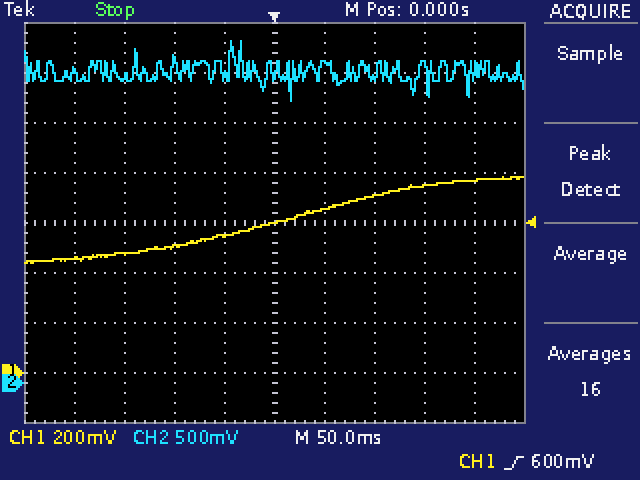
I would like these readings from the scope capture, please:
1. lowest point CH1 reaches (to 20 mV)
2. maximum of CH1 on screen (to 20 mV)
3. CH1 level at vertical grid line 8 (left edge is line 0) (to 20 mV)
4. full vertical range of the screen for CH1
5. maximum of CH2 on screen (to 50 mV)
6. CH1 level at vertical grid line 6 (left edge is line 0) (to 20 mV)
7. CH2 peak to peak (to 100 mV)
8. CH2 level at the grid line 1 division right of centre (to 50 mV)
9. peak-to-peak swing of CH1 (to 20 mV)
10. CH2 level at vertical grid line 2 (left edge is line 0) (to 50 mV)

440 mV
780 mV
740 mV
1.6 V
3.40 V
660 mV
600 mV
3.20 V
340 mV
3.05 V
